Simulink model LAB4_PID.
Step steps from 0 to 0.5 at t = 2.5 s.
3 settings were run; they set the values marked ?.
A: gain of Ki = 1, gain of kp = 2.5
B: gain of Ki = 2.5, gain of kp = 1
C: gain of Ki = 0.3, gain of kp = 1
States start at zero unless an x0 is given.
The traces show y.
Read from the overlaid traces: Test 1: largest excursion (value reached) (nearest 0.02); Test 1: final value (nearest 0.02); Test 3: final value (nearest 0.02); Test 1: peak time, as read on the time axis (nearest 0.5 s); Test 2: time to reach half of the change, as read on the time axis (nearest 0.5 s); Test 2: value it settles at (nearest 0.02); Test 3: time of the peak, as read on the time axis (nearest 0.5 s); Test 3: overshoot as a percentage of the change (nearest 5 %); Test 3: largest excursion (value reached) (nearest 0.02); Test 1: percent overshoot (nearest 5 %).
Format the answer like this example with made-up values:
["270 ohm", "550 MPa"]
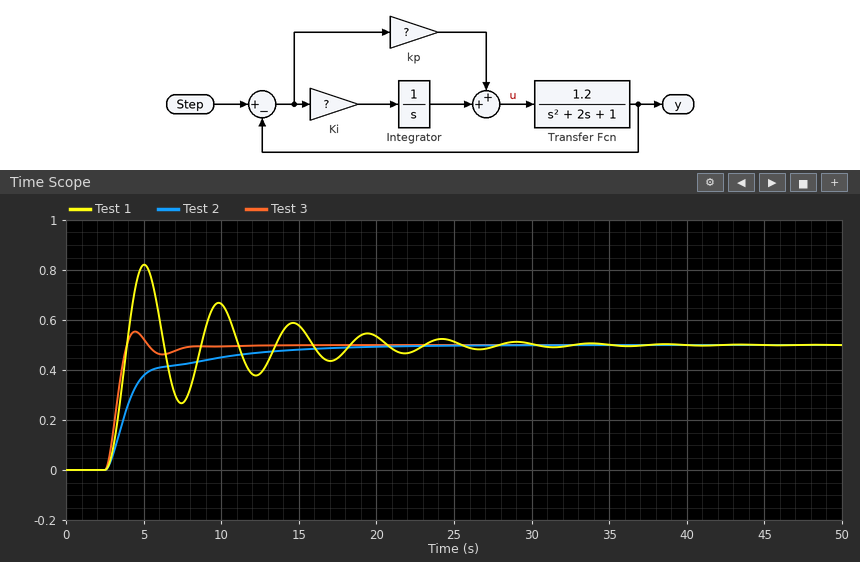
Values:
["0.82", "0.50", "0.50", "5.0 s", "4.0 s", "0.50", "4.5 s", "10 %", "0.56", "65 %"]
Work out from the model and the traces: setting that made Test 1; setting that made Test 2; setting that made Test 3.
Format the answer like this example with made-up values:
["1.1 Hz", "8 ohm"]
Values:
["B", "C", "A"]
